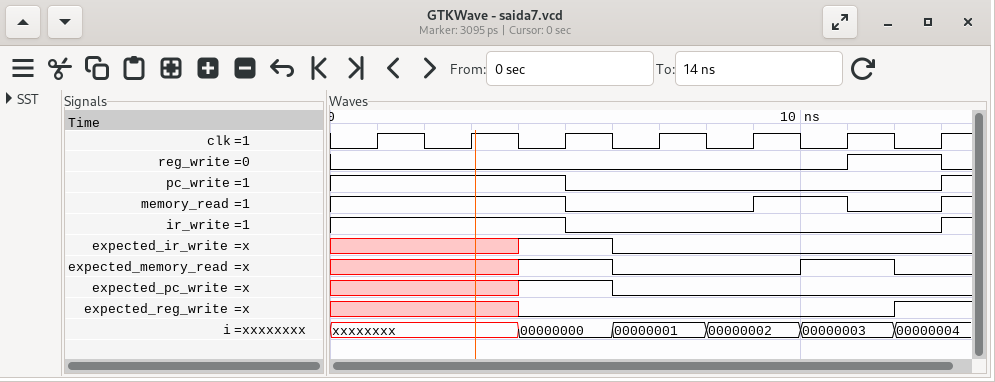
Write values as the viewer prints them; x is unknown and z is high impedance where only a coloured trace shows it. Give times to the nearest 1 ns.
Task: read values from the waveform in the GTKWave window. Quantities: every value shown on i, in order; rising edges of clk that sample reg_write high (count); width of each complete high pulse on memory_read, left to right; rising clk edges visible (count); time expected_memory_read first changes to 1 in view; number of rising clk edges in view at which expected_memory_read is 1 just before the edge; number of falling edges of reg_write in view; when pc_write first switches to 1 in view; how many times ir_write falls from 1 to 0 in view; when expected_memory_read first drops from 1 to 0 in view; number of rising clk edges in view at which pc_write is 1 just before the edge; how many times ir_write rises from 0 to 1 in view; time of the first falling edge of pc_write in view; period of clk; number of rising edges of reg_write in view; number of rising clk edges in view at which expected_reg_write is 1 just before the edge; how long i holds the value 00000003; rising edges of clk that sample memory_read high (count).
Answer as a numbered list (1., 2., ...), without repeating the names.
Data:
1. xxxxxxxx, 00000000, 00000001, 00000002, 00000003, 00000004
2. 1
3. 2 ns
4. 7
5. 4 ns
6. 2
7. 1
8. 13 ns
9. 1
10. 6 ns
11. 3
12. 1
13. 5 ns
14. 2 ns
15. 1
16. 1
17. 2 ns
18. 4
